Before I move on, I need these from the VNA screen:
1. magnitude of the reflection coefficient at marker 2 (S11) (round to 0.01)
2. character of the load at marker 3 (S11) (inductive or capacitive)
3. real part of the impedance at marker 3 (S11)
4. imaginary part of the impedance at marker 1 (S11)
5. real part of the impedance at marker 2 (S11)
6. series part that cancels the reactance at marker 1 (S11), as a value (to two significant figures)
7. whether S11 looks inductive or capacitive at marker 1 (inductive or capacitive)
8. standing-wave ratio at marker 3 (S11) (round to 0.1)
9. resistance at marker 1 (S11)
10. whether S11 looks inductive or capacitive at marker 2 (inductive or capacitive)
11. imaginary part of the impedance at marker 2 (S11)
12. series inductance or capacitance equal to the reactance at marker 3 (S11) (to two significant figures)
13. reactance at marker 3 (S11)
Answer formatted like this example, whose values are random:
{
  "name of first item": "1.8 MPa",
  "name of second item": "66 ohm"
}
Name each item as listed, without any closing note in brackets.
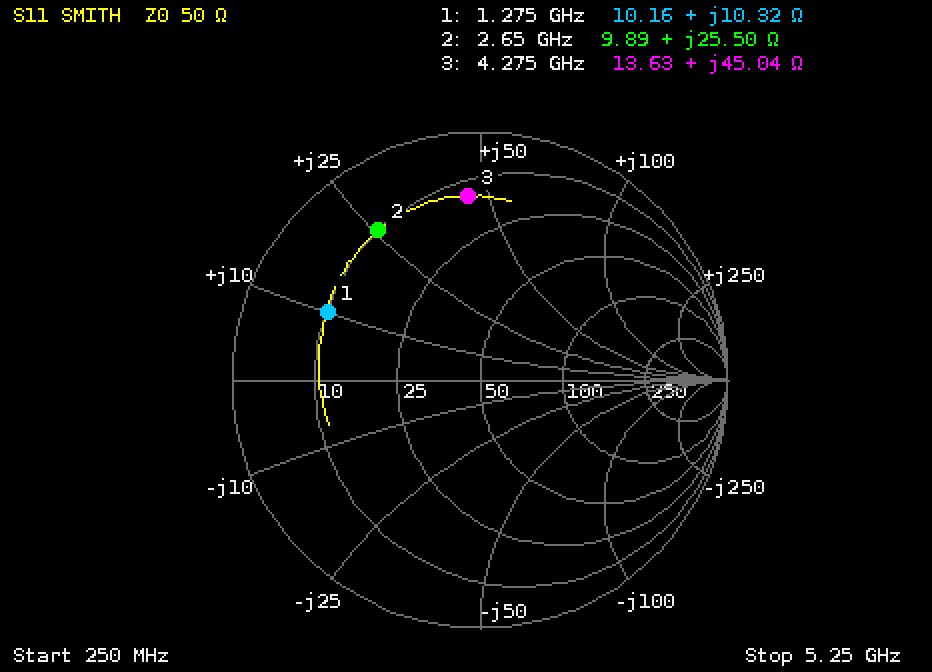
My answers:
{
  "magnitude of the reflection coefficient at marker 2 (S11)": "0.73",
  "character of the load at marker 3 (S11)": "inductive",
  "real part of the impedance at marker 3": "13.63 Ω",
  "imaginary part of the impedance at marker 1": "+10.32 Ω",
  "real part of the impedance at marker 2": "9.89 Ω",
  "series part that cancels the reactance at marker 1 (S11), as a value": "12 pF",
  "whether S11 looks inductive or capacitive at marker 1": "inductive",
  "standing-wave ratio at marker 3 (S11)": "6.8",
  "resistance at marker 1": "10.16 Ω",
  "whether S11 looks inductive or capacitive at marker 2": "inductive",
  "imaginary part of the impedance at marker 2": "+25.50 Ω",
  "series inductance or capacitance equal to the reactance at marker 3 (S11)": "1.7 nH",
  "reactance at marker 3": "+45.04 Ω"
}
